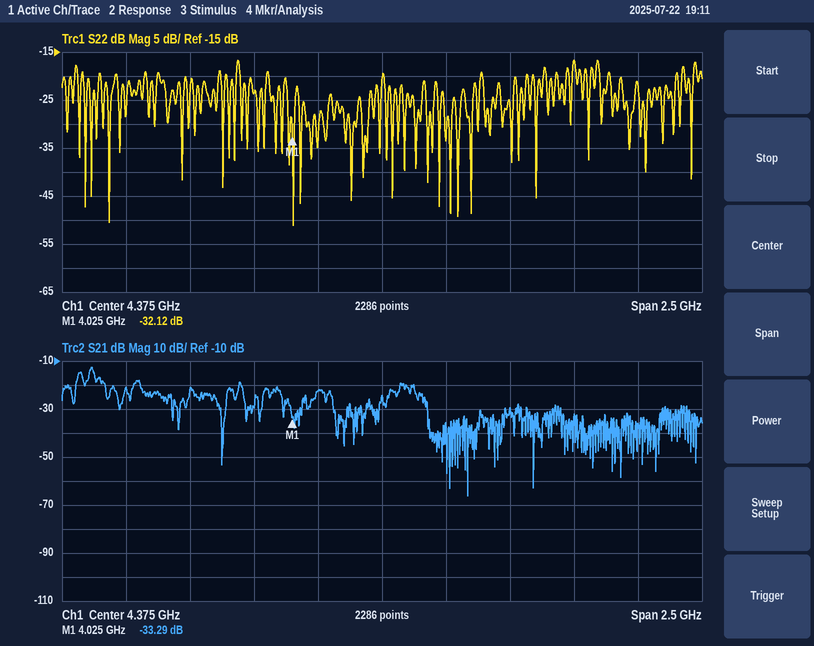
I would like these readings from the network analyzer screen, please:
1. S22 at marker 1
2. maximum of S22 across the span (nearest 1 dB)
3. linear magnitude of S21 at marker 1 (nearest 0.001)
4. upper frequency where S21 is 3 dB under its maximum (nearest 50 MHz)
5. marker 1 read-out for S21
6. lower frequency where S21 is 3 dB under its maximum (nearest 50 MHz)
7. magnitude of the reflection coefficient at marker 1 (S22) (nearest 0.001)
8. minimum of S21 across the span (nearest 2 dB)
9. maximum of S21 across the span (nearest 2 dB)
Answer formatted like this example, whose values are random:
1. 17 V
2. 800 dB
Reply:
1. -32.12 dB
2. -17 dB
3. 0.022
4. 3.25 GHz
5. -33.29 dB
6. 3.25 GHz
7. 0.025
8. -66 dB
9. -12 dB
